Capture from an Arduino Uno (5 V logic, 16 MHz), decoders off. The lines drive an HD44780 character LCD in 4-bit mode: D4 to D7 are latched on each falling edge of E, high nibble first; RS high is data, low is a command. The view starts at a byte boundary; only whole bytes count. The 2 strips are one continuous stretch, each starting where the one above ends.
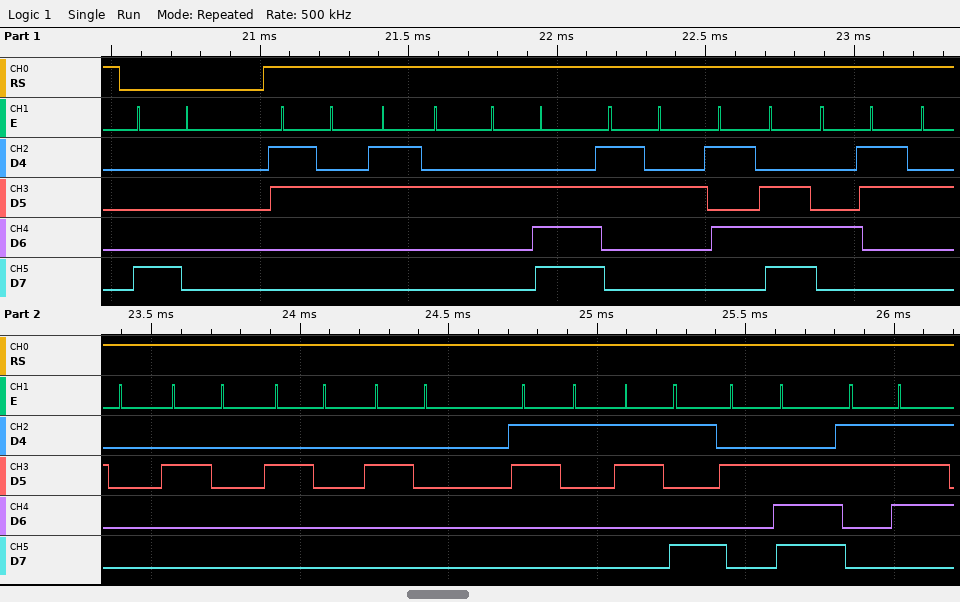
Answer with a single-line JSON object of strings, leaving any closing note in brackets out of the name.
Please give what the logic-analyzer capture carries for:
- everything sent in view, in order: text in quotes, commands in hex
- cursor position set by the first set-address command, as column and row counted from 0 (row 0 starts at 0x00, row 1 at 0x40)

{"everything sent in view, in order: text in quotes, commands in hex": "0x80 \"22.2^C    19.7\"", "cursor position set by the first set-address command, as column and row counted from 0": "column 0, row 0"}
